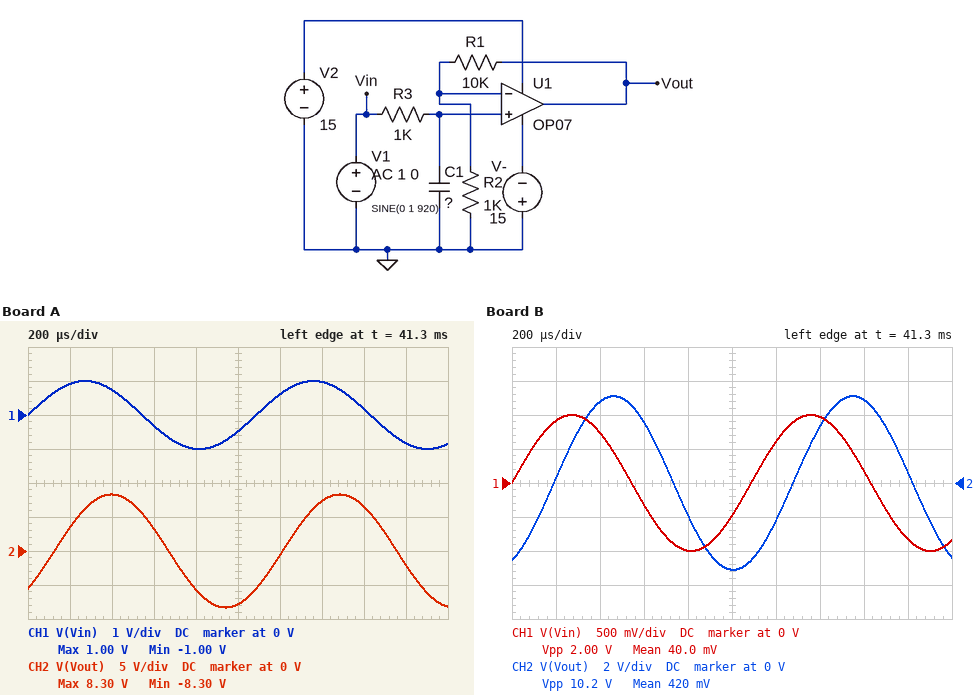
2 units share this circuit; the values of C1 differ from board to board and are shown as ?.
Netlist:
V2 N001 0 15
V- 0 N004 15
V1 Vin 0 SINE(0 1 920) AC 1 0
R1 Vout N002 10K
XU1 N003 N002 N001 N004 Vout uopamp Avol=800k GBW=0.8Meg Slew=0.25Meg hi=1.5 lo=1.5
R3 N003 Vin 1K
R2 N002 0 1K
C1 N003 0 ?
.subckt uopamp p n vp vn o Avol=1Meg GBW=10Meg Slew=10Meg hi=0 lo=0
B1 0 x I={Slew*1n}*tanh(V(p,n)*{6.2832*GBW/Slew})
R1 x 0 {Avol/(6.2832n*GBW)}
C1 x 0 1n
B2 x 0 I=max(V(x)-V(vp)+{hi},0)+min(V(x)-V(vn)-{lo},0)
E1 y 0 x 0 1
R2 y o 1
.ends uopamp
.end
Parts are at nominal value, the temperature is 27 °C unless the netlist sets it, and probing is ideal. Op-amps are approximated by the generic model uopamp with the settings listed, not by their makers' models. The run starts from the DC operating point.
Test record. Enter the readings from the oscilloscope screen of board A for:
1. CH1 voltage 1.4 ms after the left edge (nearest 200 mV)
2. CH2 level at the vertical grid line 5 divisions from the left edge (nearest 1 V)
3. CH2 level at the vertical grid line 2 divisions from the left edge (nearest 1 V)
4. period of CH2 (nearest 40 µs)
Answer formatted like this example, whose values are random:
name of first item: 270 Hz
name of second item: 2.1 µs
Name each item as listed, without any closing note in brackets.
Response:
CH1 voltage 1.4 ms after the left edge: 1.0 V
CH2 level at the vertical grid line 5 divisions from the left edge: -8 V
CH2 level at the vertical grid line 2 divisions from the left edge: 8 V
period of CH2: 1.08 ms
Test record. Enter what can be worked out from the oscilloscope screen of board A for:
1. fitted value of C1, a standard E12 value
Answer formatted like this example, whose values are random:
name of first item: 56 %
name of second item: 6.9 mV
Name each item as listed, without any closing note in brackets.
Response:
fitted value of C1, a standard E12 value: 150 nF
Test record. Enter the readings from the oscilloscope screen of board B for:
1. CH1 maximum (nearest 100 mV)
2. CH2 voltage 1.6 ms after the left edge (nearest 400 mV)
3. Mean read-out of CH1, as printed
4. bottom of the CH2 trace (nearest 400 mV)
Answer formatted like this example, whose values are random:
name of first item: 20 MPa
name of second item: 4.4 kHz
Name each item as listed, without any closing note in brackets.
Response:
CH1 maximum: 1.0 V
CH2 voltage 1.6 ms after the left edge: 4.8 V
Mean read-out of CH1, as printed: 40.0 mV
bottom of the CH2 trace: -5.2 V
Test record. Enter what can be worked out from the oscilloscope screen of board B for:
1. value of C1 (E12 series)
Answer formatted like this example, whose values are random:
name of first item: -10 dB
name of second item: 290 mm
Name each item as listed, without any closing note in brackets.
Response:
value of C1: 330 nF
